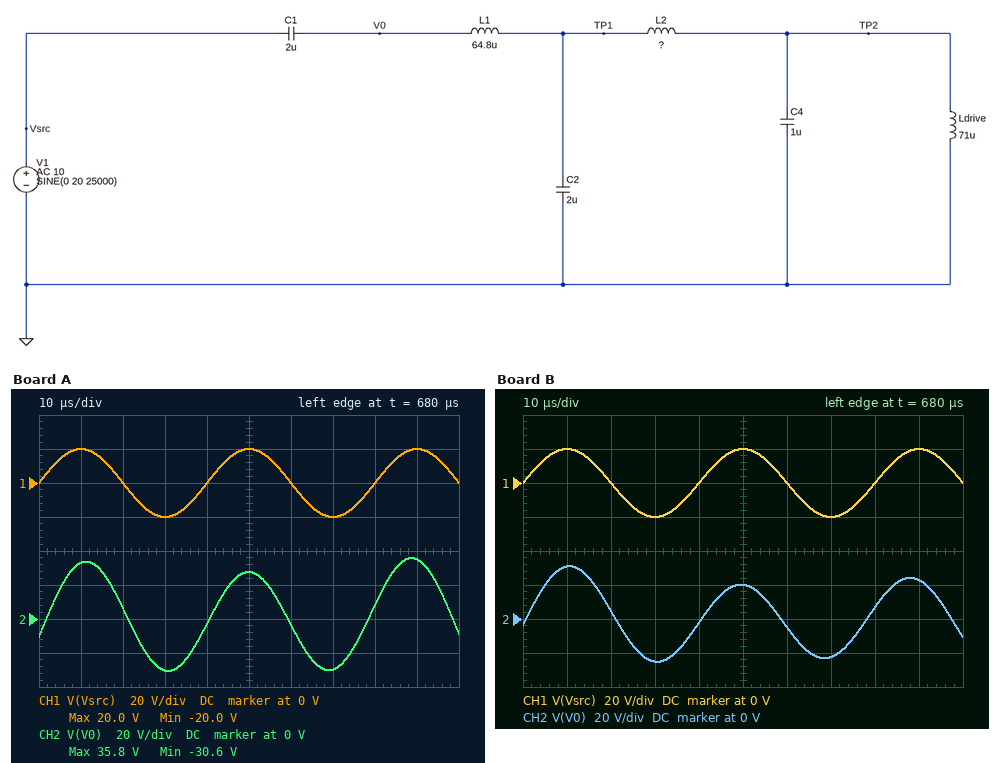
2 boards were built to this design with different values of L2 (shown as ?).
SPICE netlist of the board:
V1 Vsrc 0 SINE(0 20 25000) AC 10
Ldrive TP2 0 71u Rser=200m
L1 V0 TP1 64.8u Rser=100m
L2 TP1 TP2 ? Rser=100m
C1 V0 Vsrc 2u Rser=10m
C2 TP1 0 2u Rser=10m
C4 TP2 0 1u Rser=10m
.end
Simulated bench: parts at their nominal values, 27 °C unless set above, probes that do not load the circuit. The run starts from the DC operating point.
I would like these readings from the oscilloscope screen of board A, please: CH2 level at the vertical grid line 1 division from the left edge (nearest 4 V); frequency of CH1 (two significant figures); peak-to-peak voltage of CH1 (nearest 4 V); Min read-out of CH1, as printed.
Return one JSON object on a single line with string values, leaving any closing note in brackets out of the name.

{"CH2 level at the vertical grid line 1 division from the left edge": "32 V", "frequency of CH1": "25 kHz", "peak-to-peak voltage of CH1": "40 V", "Min read-out of CH1, as printed": "-20.0 V"}
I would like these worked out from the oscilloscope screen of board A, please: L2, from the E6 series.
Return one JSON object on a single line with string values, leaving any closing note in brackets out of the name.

{"L2, from the E6 series": "470 µH"}
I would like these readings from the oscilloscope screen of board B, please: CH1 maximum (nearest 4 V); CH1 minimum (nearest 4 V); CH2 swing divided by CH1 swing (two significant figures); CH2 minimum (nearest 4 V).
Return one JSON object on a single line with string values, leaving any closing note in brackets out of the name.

{"CH1 maximum": "20 V", "CH1 minimum": "-20 V", "CH2 swing divided by CH1 swing": "1.4", "CH2 minimum": "-24 V"}
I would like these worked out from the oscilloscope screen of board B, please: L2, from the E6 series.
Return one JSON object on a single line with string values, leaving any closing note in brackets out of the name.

{"L2, from the E6 series": "100 µH"}
